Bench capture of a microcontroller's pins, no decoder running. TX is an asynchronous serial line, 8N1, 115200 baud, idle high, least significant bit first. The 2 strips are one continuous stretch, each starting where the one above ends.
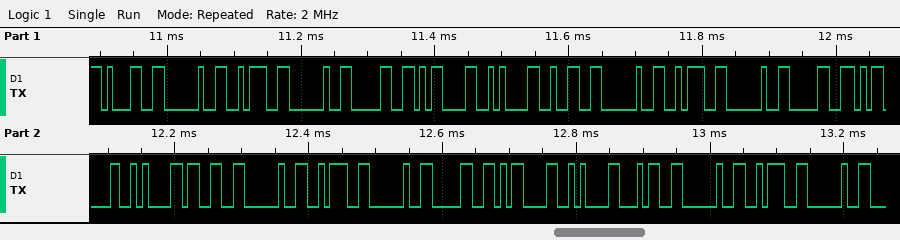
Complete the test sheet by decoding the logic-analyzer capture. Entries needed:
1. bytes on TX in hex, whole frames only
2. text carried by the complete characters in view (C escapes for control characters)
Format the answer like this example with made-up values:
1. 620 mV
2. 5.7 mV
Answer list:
1. 31 20 3A 20 30 0D 0A 32 20 3A 20 30 0D 0A 33 20 3A 20 30 0D 0A 34 20 3A 20
2. "1 : 0\r\n2 : 0\r\n3 : 0\r\n4 : "
